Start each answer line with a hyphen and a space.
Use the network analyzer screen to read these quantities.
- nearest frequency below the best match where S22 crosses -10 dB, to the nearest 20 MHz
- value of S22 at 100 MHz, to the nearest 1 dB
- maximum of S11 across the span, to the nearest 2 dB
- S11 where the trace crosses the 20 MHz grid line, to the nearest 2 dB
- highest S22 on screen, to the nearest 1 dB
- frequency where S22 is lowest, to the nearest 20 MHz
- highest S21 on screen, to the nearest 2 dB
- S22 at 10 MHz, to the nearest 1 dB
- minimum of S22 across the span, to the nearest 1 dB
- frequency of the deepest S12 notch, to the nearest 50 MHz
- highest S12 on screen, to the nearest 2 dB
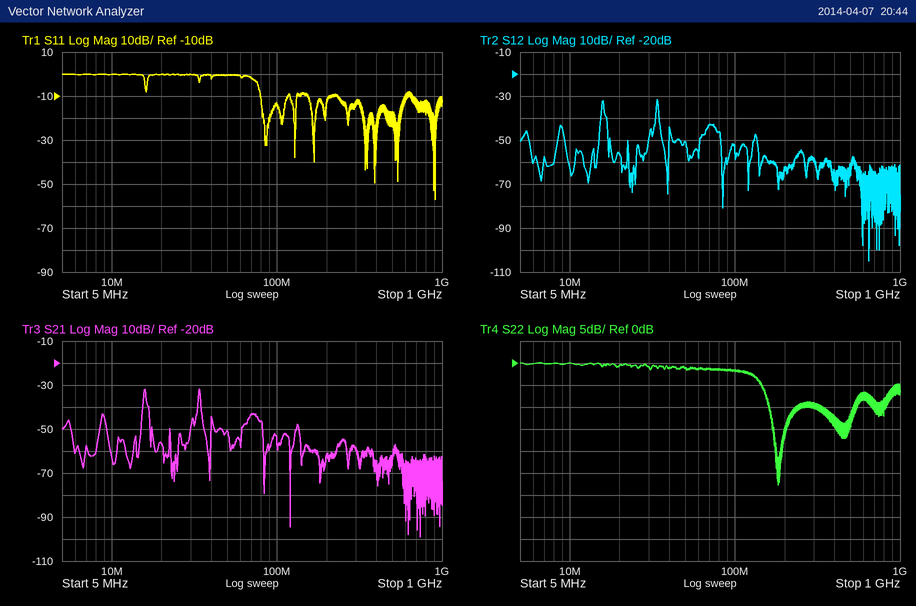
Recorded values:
- 160 MHz
- -2 dB
- 0 dB
- 0 dB
- 0 dB
- 180 MHz
- -32 dB
- 0 dB
- -28 dB
- 650 MHz
- -32 dB
